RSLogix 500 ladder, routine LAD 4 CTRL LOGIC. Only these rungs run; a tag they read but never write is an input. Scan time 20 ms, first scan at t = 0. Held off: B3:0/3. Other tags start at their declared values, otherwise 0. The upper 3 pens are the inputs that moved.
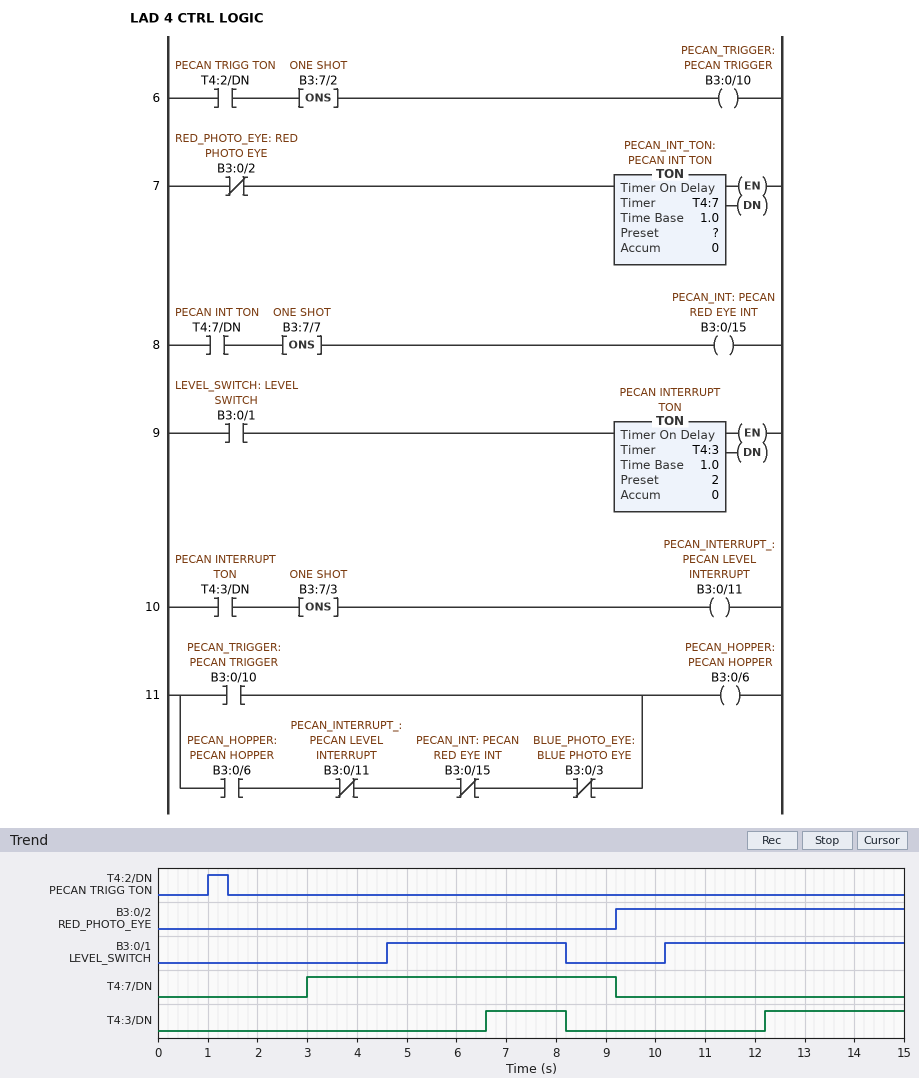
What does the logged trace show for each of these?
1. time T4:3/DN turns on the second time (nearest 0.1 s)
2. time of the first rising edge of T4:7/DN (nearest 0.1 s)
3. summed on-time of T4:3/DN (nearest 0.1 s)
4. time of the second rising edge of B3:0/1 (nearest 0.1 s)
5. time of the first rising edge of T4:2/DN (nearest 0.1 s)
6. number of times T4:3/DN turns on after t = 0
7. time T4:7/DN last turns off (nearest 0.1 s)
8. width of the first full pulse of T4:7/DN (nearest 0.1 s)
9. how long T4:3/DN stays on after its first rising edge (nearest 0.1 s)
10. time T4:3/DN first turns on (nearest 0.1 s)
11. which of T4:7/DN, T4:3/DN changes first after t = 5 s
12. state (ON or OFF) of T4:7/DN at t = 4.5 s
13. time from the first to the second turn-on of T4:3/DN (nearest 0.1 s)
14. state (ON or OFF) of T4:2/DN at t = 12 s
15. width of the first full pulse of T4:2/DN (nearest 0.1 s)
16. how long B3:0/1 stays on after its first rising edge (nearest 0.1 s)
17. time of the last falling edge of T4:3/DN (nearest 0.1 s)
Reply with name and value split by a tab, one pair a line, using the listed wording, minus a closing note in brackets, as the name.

time T4:3/DN turns on the second time	12.2 s
time of the first rising edge of T4:7/DN	3.0 s
summed on-time of T4:3/DN	4.4 s
time of the second rising edge of B3:0/1	10.2 s
time of the first rising edge of T4:2/DN	1.0 s
number of times T4:3/DN turns on after t = 0	2
time T4:7/DN last turns off	9.2 s
width of the first full pulse of T4:7/DN	6.2 s
how long T4:3/DN stays on after its first rising edge	1.6 s
time T4:3/DN first turns on	6.6 s
which of T4:7/DN, T4:3/DN changes first after t = 5 s	T4:3/DN
state (ON or OFF) of T4:7/DN at t = 4.5 s	ON
time from the first to the second turn-on of T4:3/DN	5.6 s
state (ON or OFF) of T4:2/DN at t = 12 s	OFF
width of the first full pulse of T4:2/DN	0.4 s
how long B3:0/1 stays on after its first rising edge	3.6 s
time of the last falling edge of T4:3/DN	8.2 s
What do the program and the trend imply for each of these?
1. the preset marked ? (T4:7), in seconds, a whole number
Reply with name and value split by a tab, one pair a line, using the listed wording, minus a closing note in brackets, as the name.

the preset marked ? (T4:7), in seconds, a whole number	3 s
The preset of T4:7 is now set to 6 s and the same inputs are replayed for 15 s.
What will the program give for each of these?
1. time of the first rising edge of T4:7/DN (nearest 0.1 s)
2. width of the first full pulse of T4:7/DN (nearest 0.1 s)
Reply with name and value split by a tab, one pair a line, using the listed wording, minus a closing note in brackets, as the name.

time of the first rising edge of T4:7/DN	6.0 s
width of the first full pulse of T4:7/DN	3.2 s
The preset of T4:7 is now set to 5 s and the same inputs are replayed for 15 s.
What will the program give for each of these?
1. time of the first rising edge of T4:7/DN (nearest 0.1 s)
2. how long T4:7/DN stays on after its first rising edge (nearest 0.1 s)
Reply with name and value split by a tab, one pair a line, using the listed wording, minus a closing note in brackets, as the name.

time of the first rising edge of T4:7/DN	5.0 s
how long T4:7/DN stays on after its first rising edge	4.2 s
